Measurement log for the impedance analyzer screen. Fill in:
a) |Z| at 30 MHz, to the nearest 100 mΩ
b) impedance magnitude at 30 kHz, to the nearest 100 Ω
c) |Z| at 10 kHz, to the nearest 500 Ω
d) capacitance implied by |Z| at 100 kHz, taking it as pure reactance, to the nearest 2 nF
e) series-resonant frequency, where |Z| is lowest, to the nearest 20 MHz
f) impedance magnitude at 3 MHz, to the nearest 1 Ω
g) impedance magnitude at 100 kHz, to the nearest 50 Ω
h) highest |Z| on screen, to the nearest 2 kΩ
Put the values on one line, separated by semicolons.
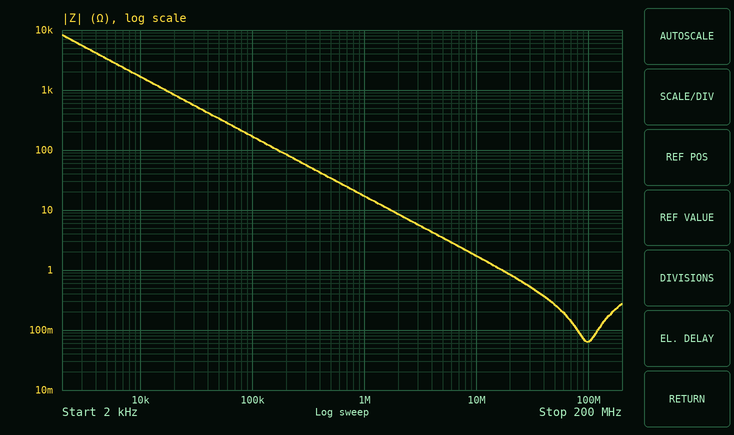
500 mΩ; 600 Ω; 1.5 kΩ; 10 nF; 100 MHz; 6 Ω; 150 Ω; 8 kΩ
